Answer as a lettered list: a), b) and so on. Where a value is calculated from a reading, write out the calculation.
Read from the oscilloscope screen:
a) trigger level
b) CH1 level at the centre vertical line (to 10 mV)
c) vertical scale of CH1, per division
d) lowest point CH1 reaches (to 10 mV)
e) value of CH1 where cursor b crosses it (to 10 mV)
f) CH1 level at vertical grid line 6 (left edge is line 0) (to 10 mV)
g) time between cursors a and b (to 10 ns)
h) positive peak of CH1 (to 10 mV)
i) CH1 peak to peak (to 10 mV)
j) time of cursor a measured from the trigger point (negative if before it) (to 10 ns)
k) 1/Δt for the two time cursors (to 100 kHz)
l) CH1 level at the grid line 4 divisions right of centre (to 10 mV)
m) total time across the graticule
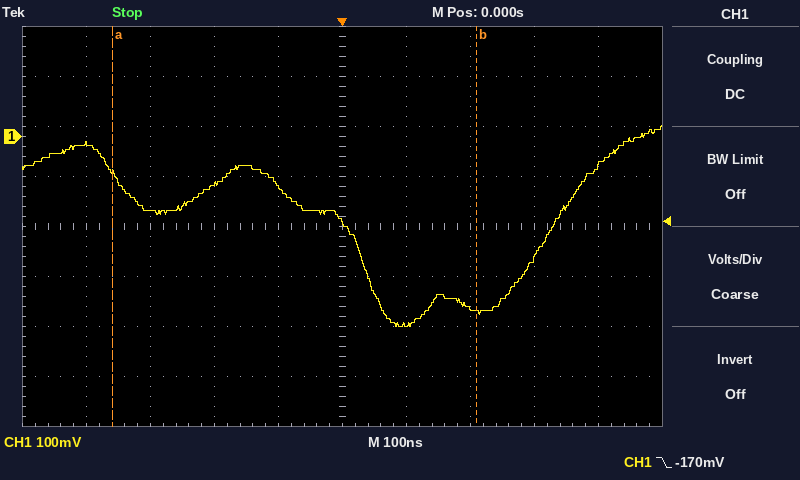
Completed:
a) -170 mV
b) -170 mV
c) 100 mV
d) -380 mV
e) -350 mV
f) -380 mV
g) 570 ns
h) 20 mV
i) 20 mV − (-380 mV) = 400 mV
j) -360 ns
k) 1 / 570 ns ≈ 1.8 MHz
l) -60 mV
m) 1 µs
